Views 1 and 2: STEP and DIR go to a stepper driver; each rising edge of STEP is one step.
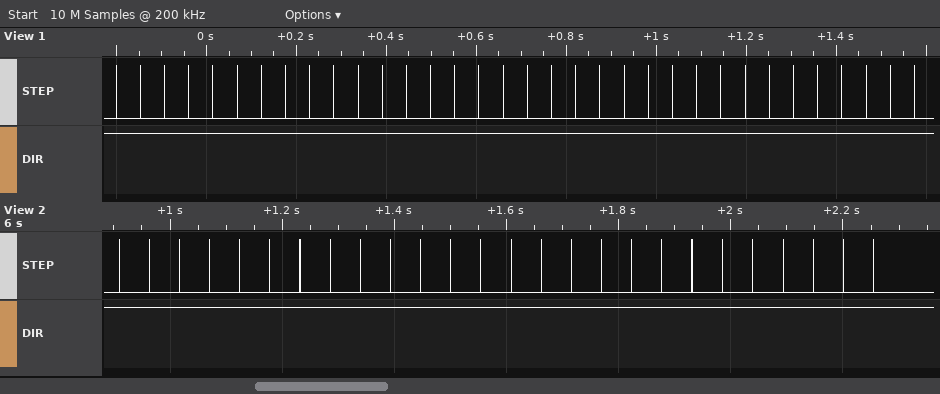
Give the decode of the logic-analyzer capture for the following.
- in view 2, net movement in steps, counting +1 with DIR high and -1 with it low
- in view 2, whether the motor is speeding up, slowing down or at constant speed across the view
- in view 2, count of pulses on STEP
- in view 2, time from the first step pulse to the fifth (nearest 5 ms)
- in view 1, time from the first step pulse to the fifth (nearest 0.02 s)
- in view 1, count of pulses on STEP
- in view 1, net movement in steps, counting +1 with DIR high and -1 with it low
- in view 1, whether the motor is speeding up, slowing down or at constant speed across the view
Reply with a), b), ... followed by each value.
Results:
a) +26
b) constant speed
c) 26
d) 215 ms
e) 0.22 s
f) 34
g) +34
h) constant speed
